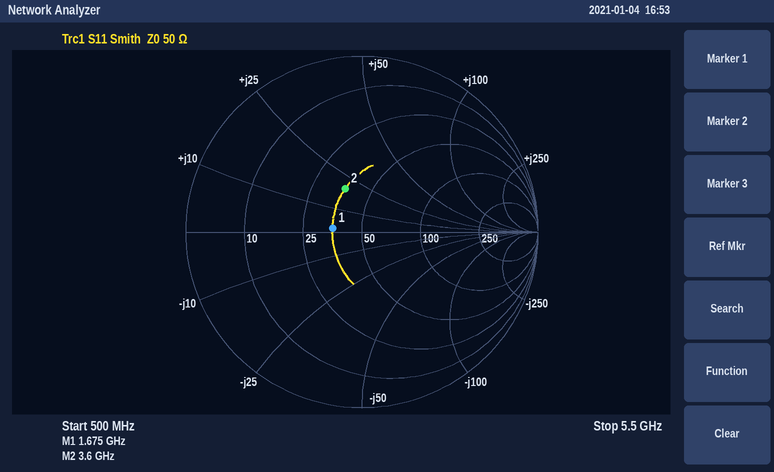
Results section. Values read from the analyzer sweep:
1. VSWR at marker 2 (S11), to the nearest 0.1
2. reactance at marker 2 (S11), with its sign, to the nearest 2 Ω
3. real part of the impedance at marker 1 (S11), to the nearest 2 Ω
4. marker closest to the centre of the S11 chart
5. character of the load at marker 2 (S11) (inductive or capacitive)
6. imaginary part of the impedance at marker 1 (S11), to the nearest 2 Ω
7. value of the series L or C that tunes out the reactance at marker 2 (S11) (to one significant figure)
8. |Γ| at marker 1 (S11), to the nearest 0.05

1.7
+20 Ω
36 Ω
marker 1
inductive
+2 Ω
2 pF
0.15
